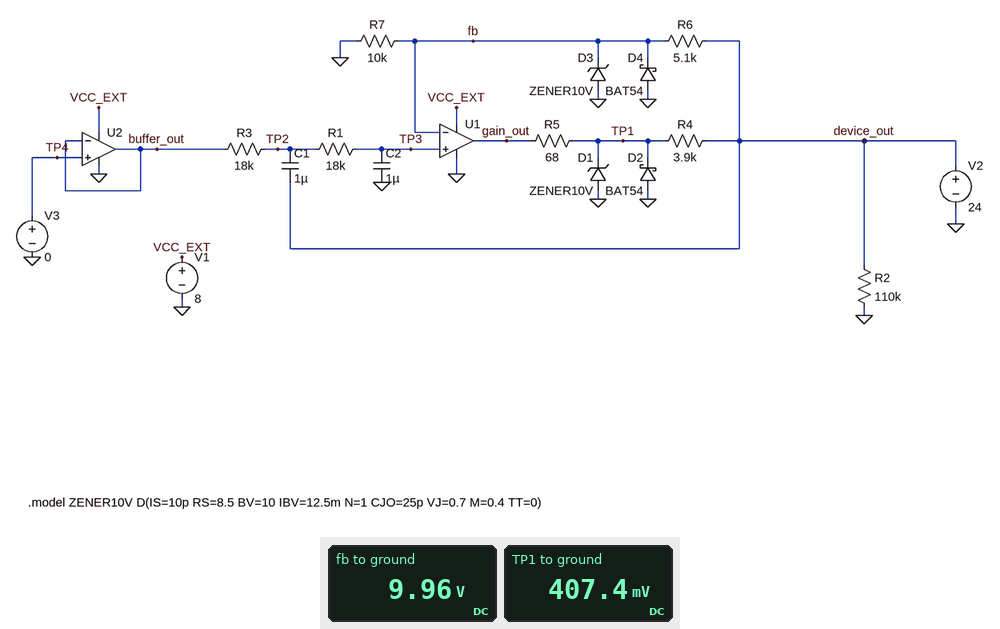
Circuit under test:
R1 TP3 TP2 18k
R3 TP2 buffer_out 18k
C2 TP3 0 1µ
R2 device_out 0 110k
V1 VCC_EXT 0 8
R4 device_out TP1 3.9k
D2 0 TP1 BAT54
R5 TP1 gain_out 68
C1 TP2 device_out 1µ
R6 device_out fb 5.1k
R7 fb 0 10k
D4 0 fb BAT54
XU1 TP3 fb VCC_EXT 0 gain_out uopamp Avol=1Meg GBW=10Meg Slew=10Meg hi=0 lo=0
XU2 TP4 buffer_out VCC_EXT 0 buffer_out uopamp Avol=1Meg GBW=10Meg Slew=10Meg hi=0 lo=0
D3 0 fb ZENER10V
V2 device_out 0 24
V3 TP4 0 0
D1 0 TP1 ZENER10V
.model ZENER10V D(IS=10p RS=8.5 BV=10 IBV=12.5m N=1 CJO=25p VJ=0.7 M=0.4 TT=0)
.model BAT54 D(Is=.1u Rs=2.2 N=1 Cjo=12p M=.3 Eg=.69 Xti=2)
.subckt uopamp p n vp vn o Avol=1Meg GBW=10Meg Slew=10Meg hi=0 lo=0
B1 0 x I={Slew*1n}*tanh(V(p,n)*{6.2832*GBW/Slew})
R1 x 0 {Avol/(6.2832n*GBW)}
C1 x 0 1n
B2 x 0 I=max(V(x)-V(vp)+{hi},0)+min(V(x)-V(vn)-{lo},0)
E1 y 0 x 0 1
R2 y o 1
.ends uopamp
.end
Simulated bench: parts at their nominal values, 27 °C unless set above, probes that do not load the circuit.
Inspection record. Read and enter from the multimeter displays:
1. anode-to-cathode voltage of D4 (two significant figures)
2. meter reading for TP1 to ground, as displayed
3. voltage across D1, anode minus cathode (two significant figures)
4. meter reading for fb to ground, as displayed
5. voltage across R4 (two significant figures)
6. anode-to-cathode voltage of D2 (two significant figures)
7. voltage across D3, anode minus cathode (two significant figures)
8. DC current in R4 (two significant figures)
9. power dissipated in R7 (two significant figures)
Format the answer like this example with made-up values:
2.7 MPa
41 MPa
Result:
-10 V
407.4 mV
-410 mV
9.96 V
24 V
-410 mV
-10 V
6.0 mA
9.9 mW
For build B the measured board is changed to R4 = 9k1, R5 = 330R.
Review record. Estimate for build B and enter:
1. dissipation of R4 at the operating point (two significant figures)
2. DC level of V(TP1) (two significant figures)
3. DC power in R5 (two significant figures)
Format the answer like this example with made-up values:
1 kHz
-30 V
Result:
59 mW
830 mV
2.1 mW
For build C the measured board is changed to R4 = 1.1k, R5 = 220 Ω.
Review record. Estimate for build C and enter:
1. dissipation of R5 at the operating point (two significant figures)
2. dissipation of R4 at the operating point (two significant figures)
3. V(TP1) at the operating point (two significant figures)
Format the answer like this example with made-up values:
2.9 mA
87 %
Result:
73 mW
360 mW
4.0 V
